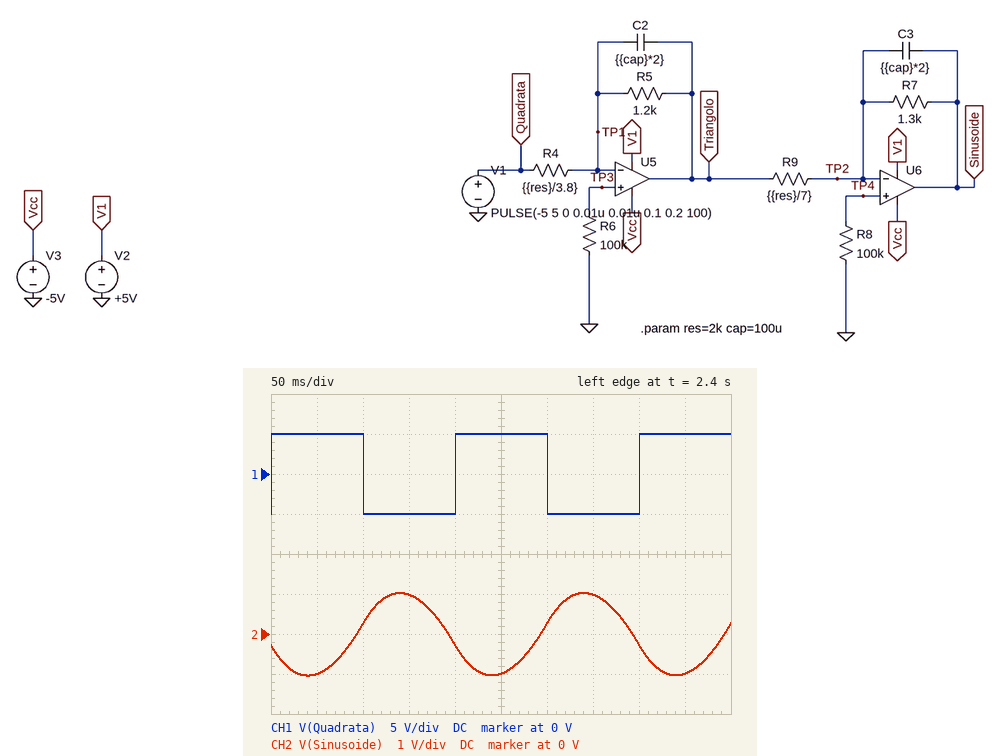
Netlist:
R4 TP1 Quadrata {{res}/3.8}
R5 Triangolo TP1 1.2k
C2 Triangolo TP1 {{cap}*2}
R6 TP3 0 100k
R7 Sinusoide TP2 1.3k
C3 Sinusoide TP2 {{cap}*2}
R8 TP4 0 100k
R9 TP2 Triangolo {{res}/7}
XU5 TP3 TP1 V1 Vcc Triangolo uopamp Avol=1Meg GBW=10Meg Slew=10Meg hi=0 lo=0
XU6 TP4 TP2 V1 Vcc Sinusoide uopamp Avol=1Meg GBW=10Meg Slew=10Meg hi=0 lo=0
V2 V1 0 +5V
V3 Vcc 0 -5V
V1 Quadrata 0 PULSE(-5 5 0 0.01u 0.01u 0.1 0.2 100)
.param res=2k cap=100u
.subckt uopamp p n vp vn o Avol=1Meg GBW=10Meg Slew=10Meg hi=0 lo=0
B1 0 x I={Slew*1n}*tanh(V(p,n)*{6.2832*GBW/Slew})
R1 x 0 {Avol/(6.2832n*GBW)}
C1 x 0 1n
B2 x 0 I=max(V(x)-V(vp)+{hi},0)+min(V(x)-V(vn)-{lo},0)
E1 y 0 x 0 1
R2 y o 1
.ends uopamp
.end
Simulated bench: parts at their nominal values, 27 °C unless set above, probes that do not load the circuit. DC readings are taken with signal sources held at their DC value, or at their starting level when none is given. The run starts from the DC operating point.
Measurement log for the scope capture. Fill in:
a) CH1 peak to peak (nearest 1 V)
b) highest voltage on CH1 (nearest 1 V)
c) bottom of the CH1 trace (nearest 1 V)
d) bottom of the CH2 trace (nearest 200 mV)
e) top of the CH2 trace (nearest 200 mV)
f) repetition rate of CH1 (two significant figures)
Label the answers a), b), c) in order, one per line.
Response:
a) 10 V
b) 5 V
c) -5 V
d) -1.0 V
e) 1.0 V
f) 5.0 Hz
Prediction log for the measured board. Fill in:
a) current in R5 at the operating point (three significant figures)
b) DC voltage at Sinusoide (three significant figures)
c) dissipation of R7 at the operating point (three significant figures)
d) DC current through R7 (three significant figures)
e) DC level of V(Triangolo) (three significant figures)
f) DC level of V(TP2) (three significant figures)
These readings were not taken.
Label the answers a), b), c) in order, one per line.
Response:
a) 5.79 mA
b) -5.00 V
c) 51.7 mW
d) 6.31 mA
e) 5.00 V
f) 3.20 V
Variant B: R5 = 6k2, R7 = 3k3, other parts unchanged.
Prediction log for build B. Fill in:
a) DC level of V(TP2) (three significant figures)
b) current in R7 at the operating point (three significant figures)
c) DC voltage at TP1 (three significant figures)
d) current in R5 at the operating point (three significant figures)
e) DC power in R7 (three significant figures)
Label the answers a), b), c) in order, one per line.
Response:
a) 4.21 V
b) 2.79 mA
c) -4.22 V
d) 1.49 mA
e) 25.7 mW
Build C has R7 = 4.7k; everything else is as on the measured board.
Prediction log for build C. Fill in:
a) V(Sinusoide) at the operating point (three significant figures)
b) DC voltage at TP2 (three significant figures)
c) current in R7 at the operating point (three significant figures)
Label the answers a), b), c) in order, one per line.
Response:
a) -5.01 V
b) 4.43 V
c) 2.01 mA
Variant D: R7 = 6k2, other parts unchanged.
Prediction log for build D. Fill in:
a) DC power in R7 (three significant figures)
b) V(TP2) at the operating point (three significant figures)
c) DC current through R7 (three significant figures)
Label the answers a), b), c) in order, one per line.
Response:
a) 14.8 mW
b) 4.56 V
c) 1.54 mA
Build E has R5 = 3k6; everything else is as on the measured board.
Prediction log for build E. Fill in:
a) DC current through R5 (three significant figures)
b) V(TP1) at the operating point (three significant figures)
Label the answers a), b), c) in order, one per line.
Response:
a) 2.42 mA
b) -3.72 V
